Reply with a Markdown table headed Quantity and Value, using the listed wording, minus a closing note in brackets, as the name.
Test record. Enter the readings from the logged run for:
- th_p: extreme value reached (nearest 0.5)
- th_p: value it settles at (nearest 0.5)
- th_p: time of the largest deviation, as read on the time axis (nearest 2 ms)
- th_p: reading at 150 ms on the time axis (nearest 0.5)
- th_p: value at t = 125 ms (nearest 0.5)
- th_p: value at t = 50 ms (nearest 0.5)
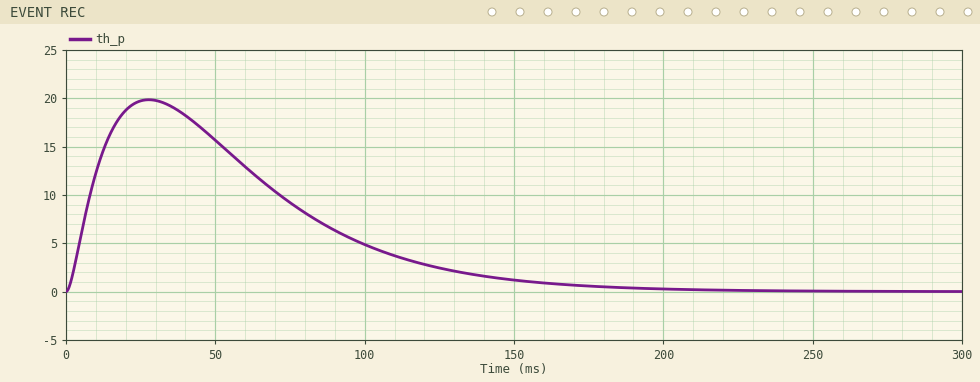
| Quantity | Value |
|---|---|
| th_p: extreme value reached | 20.0 |
| th_p: value it settles at | 0.0 |
| th_p: time of the largest deviation, as read on the time axis | 28 ms |
| th_p: reading at 150 ms on the time axis | 1.0 |
| th_p: value at t = 125 ms | 2.5 |
| th_p: value at t = 50 ms | 15.5 |
